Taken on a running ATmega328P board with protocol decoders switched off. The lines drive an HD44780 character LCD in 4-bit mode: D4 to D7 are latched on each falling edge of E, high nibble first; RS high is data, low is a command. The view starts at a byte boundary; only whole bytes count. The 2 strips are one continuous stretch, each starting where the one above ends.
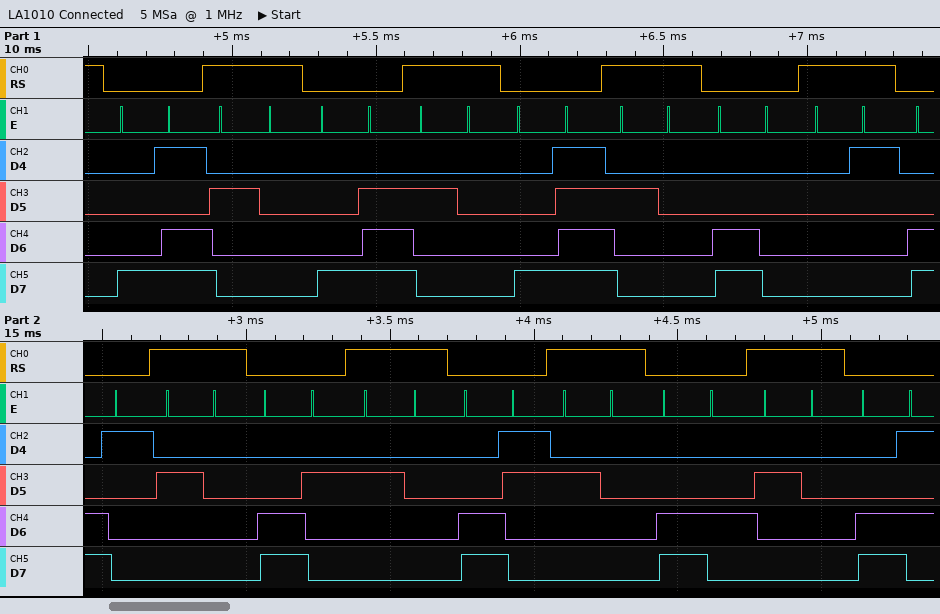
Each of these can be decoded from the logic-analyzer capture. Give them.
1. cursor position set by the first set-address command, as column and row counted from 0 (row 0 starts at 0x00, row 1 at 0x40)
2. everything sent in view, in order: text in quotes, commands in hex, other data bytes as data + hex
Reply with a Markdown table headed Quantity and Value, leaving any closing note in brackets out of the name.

| Quantity | Value |
|---|---|
| cursor position set by the first set-address command, as column and row counted from 0 | column 13, row 0 |
| everything sent in view, in order: text in quotes, commands in hex, other data bytes as data + hex | 0x8D " " 0x8E " " 0x8F " " 0xC0 data 01 0xC1 " " 0xC2 " " 0xC3 " " 0xC4 " " 0xC5 |
